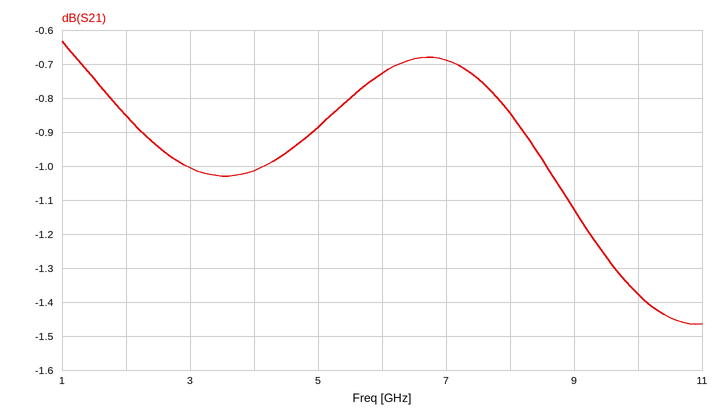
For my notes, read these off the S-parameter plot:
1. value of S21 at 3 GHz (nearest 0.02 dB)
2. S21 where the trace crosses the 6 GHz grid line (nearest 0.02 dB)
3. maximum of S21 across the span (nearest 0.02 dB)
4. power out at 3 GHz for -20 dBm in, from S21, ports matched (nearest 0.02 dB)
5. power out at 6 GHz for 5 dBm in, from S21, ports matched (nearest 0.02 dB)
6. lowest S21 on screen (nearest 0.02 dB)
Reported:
-1.00 dB
-0.72 dB
-0.64 dB
-21.00 dBm
4.28 dBm
-1.46 dB
